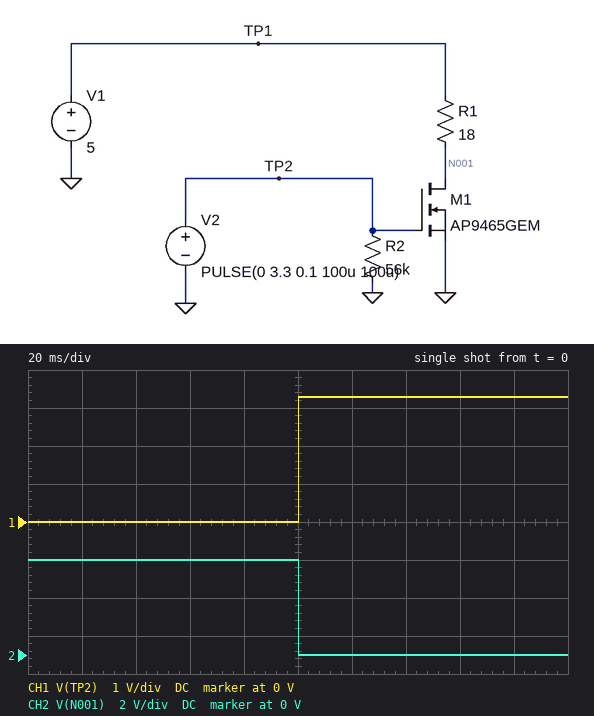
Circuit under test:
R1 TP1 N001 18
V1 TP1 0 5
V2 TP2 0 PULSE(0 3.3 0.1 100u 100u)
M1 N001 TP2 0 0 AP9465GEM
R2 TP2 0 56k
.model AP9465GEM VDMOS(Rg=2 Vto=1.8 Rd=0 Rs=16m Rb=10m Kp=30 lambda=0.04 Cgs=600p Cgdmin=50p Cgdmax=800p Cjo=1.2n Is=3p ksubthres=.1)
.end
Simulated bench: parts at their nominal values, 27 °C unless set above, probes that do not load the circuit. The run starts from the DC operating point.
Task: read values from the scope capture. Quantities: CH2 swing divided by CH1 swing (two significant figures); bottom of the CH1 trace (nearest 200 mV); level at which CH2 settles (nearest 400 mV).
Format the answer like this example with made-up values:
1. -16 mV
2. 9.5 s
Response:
1. 1.5
2. 0 V
3. 0 V
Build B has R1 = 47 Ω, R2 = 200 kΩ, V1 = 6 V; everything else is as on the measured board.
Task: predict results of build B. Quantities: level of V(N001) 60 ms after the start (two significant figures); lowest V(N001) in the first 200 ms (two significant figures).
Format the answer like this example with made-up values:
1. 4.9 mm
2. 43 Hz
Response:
1. 6.0 V
2. 4.9 mV
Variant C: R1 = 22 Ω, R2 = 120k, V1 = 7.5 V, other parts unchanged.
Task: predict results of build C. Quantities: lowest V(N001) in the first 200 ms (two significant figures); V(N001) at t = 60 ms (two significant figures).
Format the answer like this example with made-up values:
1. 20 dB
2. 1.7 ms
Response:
1. 13 mV
2. 7.5 V
